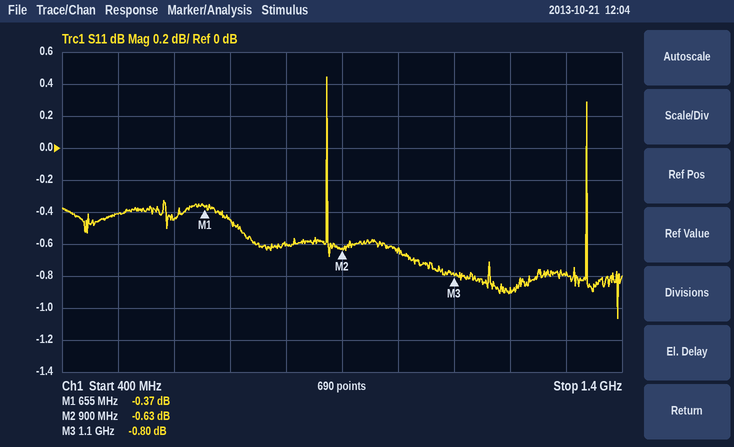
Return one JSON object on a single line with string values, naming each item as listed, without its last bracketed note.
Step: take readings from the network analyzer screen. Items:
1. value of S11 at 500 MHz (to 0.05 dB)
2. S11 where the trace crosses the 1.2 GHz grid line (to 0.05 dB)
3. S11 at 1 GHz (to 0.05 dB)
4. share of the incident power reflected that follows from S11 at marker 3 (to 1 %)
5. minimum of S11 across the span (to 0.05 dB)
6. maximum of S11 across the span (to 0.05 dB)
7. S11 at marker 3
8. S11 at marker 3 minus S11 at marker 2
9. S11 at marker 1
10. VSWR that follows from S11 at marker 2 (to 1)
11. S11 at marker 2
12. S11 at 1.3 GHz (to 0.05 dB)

{"value of S11 at 500 MHz": "-0.40 dB", "S11 where the trace crosses the 1.2 GHz grid line": "-0.90 dB", "S11 at 1 GHz": "-0.65 dB", "share of the incident power reflected that follows from S11 at marker 3": "83 %", "minimum of S11 across the span": "-1.05 dB", "maximum of S11 across the span": "0.45 dB", "S11 at marker 3": "-0.80 dB", "S11 at marker 3 minus S11 at marker 2": "-0.17 dB", "S11 at marker 1": "-0.37 dB", "VSWR that follows from S11 at marker 2": "28", "S11 at marker 2": "-0.63 dB", "S11 at 1.3 GHz": "-0.80 dB"}
